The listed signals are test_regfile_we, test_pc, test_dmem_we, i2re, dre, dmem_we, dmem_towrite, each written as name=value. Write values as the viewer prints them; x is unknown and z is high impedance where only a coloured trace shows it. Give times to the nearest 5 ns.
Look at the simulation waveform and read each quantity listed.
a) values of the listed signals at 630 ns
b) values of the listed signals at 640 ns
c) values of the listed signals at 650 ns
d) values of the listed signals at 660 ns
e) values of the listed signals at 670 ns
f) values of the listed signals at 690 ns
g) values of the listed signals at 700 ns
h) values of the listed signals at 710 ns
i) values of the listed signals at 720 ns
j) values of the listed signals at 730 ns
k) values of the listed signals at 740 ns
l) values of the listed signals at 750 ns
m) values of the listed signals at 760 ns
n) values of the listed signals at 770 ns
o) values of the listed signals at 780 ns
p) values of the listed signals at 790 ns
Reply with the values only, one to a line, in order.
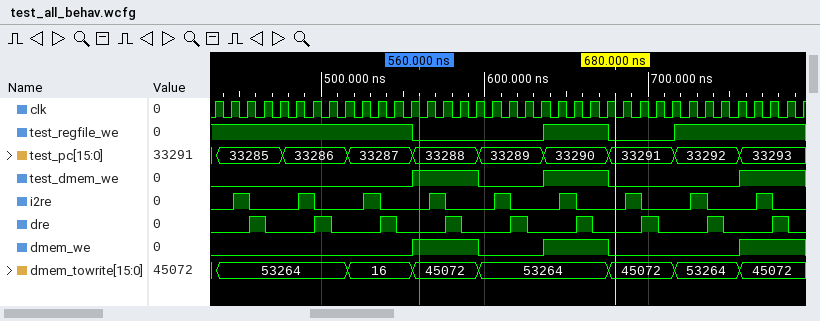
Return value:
test_regfile_we=0, test_pc=33289, test_dmem_we=0, i2re=0, dre=0, dmem_we=0, dmem_towrite=53264
test_regfile_we=1, test_pc=33290, test_dmem_we=1, i2re=0, dre=0, dmem_we=1, dmem_towrite=53264
test_regfile_we=1, test_pc=33290, test_dmem_we=1, i2re=1, dre=0, dmem_we=1, dmem_towrite=53264
test_regfile_we=1, test_pc=33290, test_dmem_we=1, i2re=0, dre=1, dmem_we=1, dmem_towrite=53264
test_regfile_we=1, test_pc=33290, test_dmem_we=1, i2re=0, dre=0, dmem_we=1, dmem_towrite=53264
test_regfile_we=0, test_pc=33291, test_dmem_we=0, i2re=1, dre=0, dmem_we=0, dmem_towrite=45072
test_regfile_we=0, test_pc=33291, test_dmem_we=0, i2re=0, dre=1, dmem_we=0, dmem_towrite=45072
test_regfile_we=0, test_pc=33291, test_dmem_we=0, i2re=0, dre=0, dmem_we=0, dmem_towrite=45072
test_regfile_we=1, test_pc=33292, test_dmem_we=0, i2re=0, dre=0, dmem_we=0, dmem_towrite=53264
test_regfile_we=1, test_pc=33292, test_dmem_we=0, i2re=1, dre=0, dmem_we=0, dmem_towrite=53264
test_regfile_we=1, test_pc=33292, test_dmem_we=0, i2re=0, dre=1, dmem_we=0, dmem_towrite=53264
test_regfile_we=1, test_pc=33292, test_dmem_we=0, i2re=0, dre=0, dmem_we=0, dmem_towrite=53264
test_regfile_we=1, test_pc=33293, test_dmem_we=1, i2re=0, dre=0, dmem_we=1, dmem_towrite=45072
test_regfile_we=1, test_pc=33293, test_dmem_we=1, i2re=1, dre=0, dmem_we=1, dmem_towrite=45072
test_regfile_we=1, test_pc=33293, test_dmem_we=1, i2re=0, dre=1, dmem_we=1, dmem_towrite=45072
test_regfile_we=1, test_pc=33293, test_dmem_we=1, i2re=0, dre=0, dmem_we=1, dmem_towrite=45072
